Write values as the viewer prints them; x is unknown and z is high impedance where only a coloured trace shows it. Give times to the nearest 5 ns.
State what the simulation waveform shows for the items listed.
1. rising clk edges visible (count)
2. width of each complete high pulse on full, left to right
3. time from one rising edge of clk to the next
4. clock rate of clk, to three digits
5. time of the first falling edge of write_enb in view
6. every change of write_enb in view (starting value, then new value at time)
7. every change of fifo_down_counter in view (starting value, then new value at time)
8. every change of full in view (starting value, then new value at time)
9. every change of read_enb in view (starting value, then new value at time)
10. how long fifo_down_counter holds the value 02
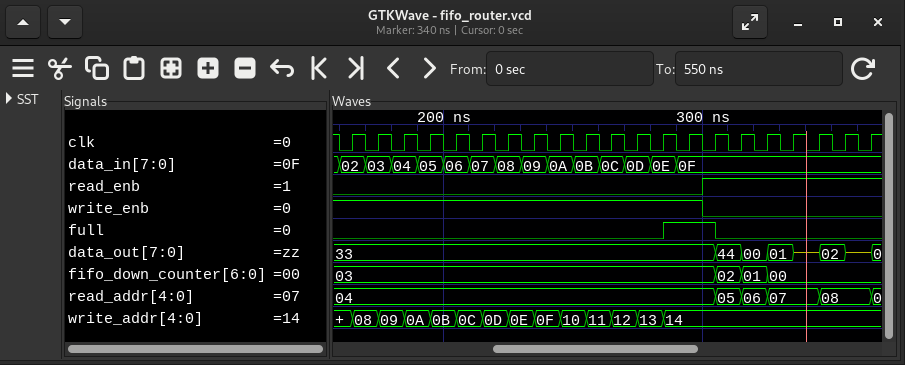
21
20 ns
10 ns
100 MHz
300 ns
1, 0 at 300 ns
03, 02 at 305 ns, 01 at 315 ns, 00 at 325 ns
0, 1 at 285 ns, 0 at 305 ns
0, 1 at 300 ns
10 ns
